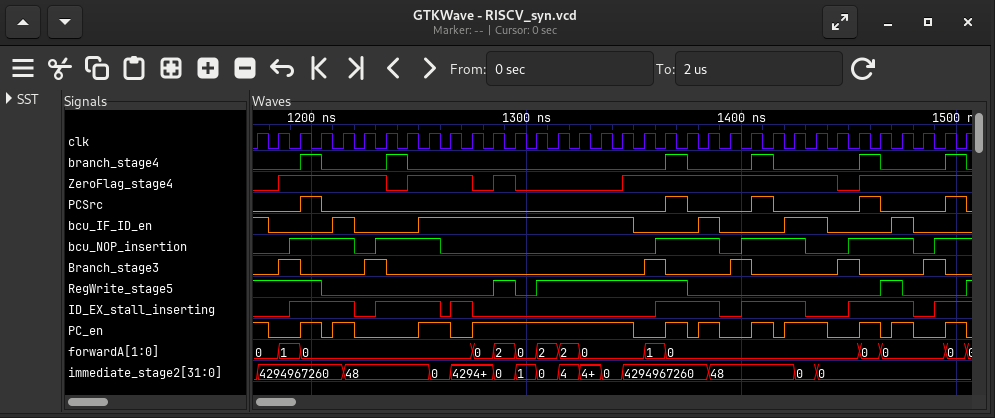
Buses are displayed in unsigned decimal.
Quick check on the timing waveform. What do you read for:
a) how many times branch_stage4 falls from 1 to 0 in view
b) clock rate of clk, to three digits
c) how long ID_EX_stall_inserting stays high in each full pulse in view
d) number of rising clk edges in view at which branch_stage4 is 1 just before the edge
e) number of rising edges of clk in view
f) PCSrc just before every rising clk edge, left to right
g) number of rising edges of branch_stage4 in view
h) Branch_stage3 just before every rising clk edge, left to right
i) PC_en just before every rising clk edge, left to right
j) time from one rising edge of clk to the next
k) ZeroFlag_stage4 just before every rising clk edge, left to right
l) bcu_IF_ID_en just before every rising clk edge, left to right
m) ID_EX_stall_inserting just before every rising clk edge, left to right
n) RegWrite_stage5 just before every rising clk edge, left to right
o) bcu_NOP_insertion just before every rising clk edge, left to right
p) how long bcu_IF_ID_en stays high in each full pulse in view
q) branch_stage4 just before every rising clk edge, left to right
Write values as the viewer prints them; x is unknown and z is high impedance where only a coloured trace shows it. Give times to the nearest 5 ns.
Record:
6
100 MHz
30 ns, 30 ns, 10 ns, 30 ns, 30 ns, 30 ns
6
34
0 0 0 1 0 0 0 0 0 0 0 0 0 0 0 0 0 0 0 0 1 0 0 0 1 0 0 0 0 1 0 0 0 1
6
0 0 1 0 0 0 1 0 0 0 0 0 0 0 0 0 0 0 0 1 0 0 0 1 0 0 0 0 1 0 0 0 1 0
1 0 0 1 1 0 0 0 1 1 0 1 1 1 1 1 1 1 0 0 1 1 0 0 1 1 1 0 0 1 1 0 0 1
10 ns
0 0 1 1 1 1 1 0 1 1 1 0 1 0 0 0 0 0 1 1 1 1 1 1 1 1 1 1 0 1 1 1 1 1
1 0 0 0 1 0 0 0 1 1 1 1 1 1 1 1 1 1 0 0 0 1 0 0 0 1 1 0 0 0 1 0 0 0
0 0 1 1 1 0 1 1 1 0 1 0 0 0 0 0 0 0 0 1 1 1 0 1 1 1 0 0 1 1 1 0 1 1
1 1 1 1 0 0 0 0 0 0 0 0 1 0 1 1 1 1 1 1 1 0 0 0 0 0 0 0 0 0 1 0 0 0
0 0 1 1 1 0 1 1 1 0 0 0 0 0 0 0 0 0 0 1 1 1 0 1 1 1 0 0 1 1 1 0 1 1
10 ns, 100 ns, 10 ns, 20 ns, 10 ns
0 0 0 1 0 0 0 1 0 0 0 0 0 0 0 0 0 0 0 0 1 0 0 0 1 0 0 0 0 1 0 0 0 1
